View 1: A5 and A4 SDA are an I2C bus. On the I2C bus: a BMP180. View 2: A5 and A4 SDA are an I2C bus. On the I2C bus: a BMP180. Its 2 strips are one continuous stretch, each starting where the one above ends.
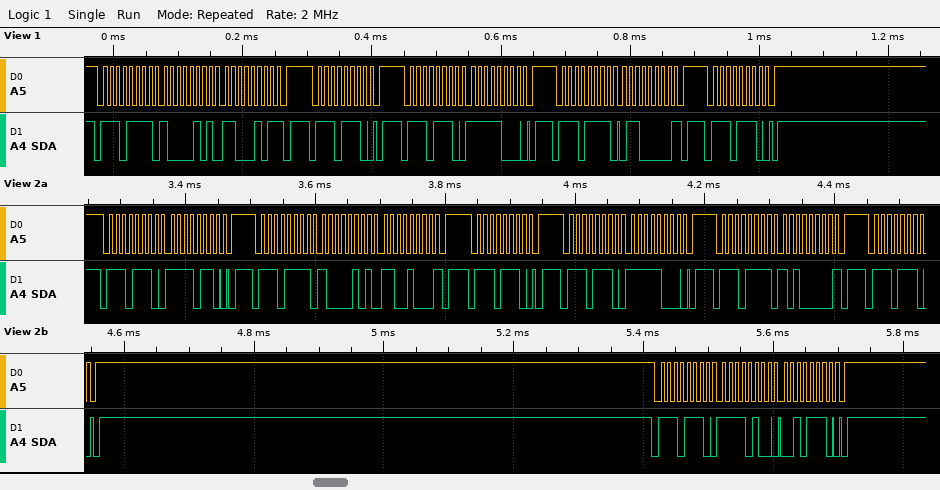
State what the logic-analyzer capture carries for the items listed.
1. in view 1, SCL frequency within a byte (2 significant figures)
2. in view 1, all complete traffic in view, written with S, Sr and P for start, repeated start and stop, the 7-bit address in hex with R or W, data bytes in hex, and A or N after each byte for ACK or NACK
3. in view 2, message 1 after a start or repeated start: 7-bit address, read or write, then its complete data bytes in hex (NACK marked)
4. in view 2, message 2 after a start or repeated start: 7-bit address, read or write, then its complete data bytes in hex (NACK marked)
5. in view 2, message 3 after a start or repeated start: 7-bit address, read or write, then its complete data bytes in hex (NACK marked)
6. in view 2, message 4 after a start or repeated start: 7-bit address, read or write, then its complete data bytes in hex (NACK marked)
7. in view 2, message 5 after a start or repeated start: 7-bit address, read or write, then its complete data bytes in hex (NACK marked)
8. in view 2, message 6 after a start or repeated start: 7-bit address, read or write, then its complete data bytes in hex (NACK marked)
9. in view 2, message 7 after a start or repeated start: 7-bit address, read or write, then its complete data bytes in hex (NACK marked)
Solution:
100 kHz
S 77R A 85 A C5 N P S 77W A P S 77W A F8 A P S 77R A 60 N P S 77W A P
0x77 write: F6
0x77 read: 85 C8 NACK
0x77 write
0x77 write: F8
0x77 read: A0 NACK
0x77 write
0x77 write: F4 2E
